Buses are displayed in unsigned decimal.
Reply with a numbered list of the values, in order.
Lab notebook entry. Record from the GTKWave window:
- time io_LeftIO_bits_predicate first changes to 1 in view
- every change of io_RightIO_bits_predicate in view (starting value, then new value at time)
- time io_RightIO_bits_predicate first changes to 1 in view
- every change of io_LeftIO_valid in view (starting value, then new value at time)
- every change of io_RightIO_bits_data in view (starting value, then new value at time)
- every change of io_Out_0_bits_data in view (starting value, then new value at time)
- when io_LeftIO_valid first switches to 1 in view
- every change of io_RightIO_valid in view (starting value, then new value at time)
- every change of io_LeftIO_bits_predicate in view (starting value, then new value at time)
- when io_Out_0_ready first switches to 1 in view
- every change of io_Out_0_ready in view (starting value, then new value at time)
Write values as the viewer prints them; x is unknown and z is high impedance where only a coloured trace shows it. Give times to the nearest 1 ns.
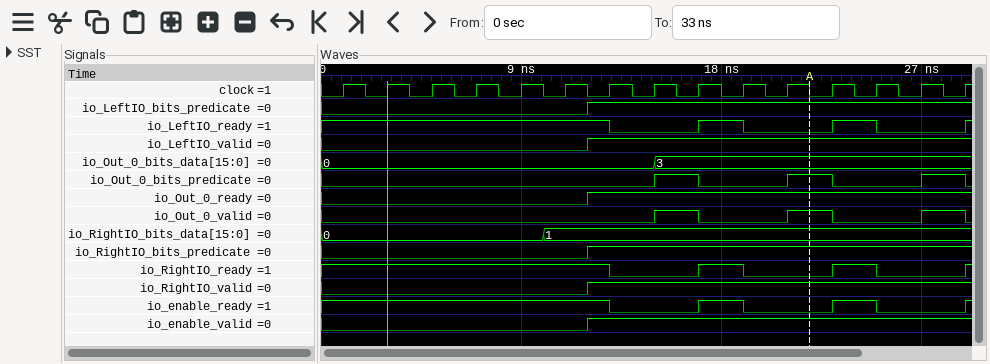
1. 12 ns
2. 0, 1 at 12 ns
3. 12 ns
4. 0, 1 at 12 ns
5. 0, 1 at 10 ns
6. 0, 3 at 15 ns
7. 12 ns
8. 0, 1 at 12 ns
9. 0, 1 at 12 ns
10. 12 ns
11. 0, 1 at 12 ns
